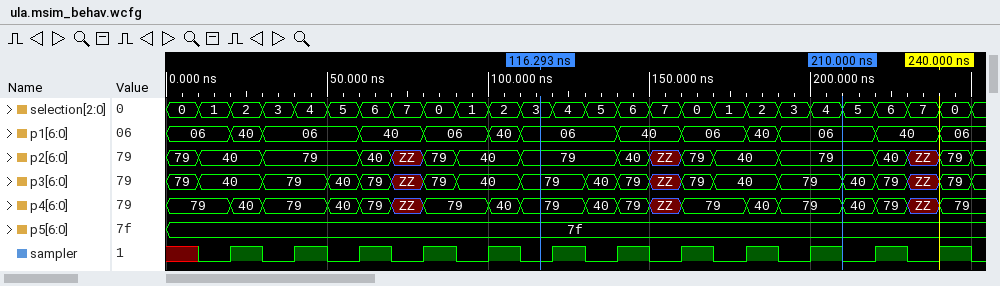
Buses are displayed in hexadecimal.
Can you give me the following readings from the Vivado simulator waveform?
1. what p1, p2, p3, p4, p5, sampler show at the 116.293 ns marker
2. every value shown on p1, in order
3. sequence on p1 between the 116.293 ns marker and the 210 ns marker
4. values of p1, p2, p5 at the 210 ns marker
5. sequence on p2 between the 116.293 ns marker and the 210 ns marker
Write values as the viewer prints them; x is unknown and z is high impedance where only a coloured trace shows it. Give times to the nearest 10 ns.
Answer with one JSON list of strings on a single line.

["p1=06, p2=79, p3=79, p4=79, p5=7f, sampler=0", "06, 40, 06, 40, 06, 40, 06, 40, 06, 40, 06, 40, 06", "06, 40, 06, 40, 06", "p1=06, p2=79, p5=7f", "79, 40, ZZ, 79, 40, 79"]
